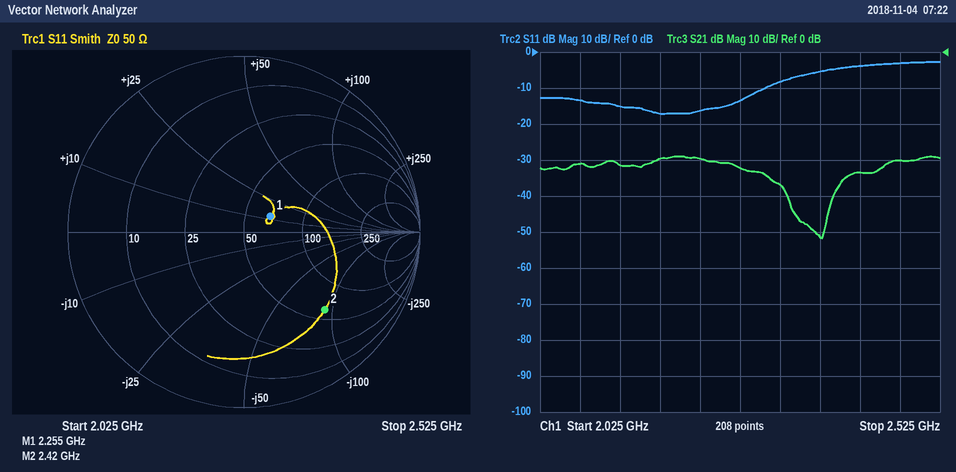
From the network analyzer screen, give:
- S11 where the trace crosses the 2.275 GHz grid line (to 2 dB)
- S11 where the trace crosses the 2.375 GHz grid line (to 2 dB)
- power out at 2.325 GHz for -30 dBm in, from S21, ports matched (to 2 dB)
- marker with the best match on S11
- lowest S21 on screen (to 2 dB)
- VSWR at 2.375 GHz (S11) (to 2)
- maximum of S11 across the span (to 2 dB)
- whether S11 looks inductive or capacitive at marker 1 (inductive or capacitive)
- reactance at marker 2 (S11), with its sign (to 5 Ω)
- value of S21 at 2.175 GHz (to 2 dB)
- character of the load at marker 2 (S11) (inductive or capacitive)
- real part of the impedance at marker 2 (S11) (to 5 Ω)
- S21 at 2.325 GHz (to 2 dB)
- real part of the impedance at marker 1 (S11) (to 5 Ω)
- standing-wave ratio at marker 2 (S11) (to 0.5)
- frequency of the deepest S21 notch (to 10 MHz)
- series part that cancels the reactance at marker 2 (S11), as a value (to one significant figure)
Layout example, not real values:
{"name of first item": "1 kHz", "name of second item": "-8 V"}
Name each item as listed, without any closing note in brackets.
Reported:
{"S11 where the trace crosses the 2.275 GHz grid line": "-14 dB", "S11 where the trace crosses the 2.375 GHz grid line": "-6 dB", "power out at 2.325 GHz for -30 dBm in, from S21, ports matched": "-66 dBm", "marker with the best match on S11": "marker 1", "lowest S21 on screen": "-52 dB", "VSWR at 2.375 GHz (S11)": "4", "maximum of S11 across the span": "-2 dB", "whether S11 looks inductive or capacitive at marker 1": "inductive", "reactance at marker 2 (S11), with its sign": "-90 Ω", "value of S21 at 2.175 GHz": "-30 dB", "character of the load at marker 2 (S11)": "capacitive", "real part of the impedance at marker 2 (S11)": "60 Ω", "S21 at 2.325 GHz": "-36 dB", "real part of the impedance at marker 1 (S11)": "65 Ω", "standing-wave ratio at marker 2 (S11)": "4.5", "frequency of the deepest S21 notch": "2.38 GHz", "series part that cancels the reactance at marker 2 (S11), as a value": "6 nH"}
